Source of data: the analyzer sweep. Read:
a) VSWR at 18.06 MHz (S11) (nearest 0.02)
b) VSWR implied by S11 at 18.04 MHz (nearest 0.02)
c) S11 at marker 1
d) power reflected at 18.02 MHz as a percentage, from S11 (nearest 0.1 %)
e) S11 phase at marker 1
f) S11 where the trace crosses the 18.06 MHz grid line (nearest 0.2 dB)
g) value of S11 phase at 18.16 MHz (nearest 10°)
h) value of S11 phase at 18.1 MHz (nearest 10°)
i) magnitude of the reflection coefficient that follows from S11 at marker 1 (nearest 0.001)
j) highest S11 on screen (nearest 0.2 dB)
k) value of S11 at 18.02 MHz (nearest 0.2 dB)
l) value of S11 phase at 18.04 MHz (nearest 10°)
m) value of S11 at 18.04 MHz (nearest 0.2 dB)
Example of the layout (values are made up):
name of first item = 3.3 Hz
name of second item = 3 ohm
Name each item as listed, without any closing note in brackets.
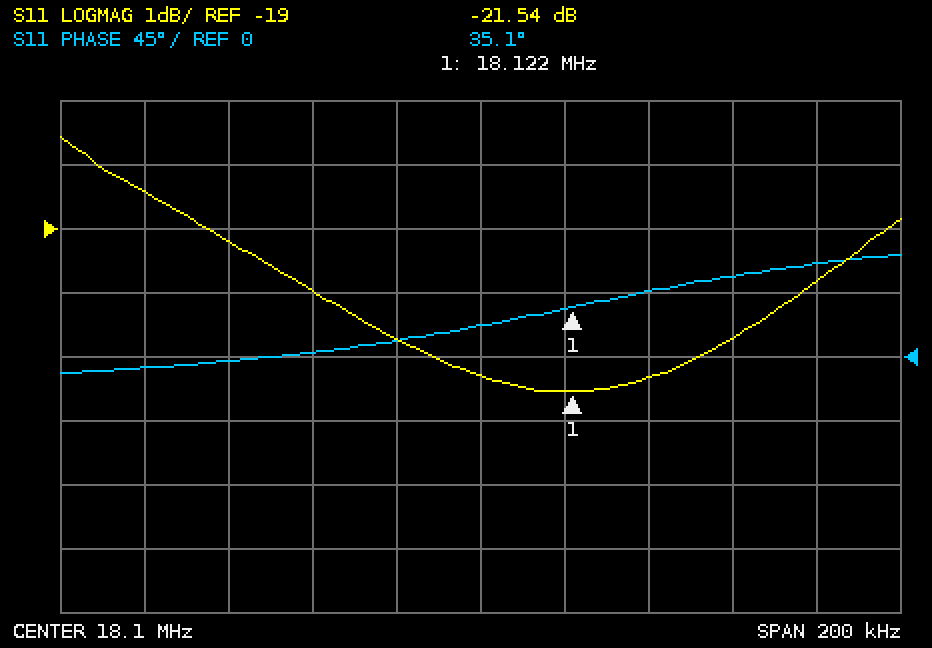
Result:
VSWR at 18.06 MHz (S11) = 1.22
VSWR implied by S11 at 18.04 MHz = 1.24
S11 at marker 1 = -21.54 dB
power reflected at 18.02 MHz as a percentage, from S11 = 1.4 %
S11 phase at marker 1 = 35.1°
S11 where the trace crosses the 18.06 MHz grid line = -20.0 dB
value of S11 phase at 18.16 MHz = 60°
value of S11 phase at 18.1 MHz = 20°
magnitude of the reflection coefficient that follows from S11 at marker 1 = 0.084
highest S11 on screen = -17.6 dB
value of S11 at 18.02 MHz = -18.4 dB
value of S11 phase at 18.04 MHz = 0°
value of S11 at 18.04 MHz = -19.2 dB
